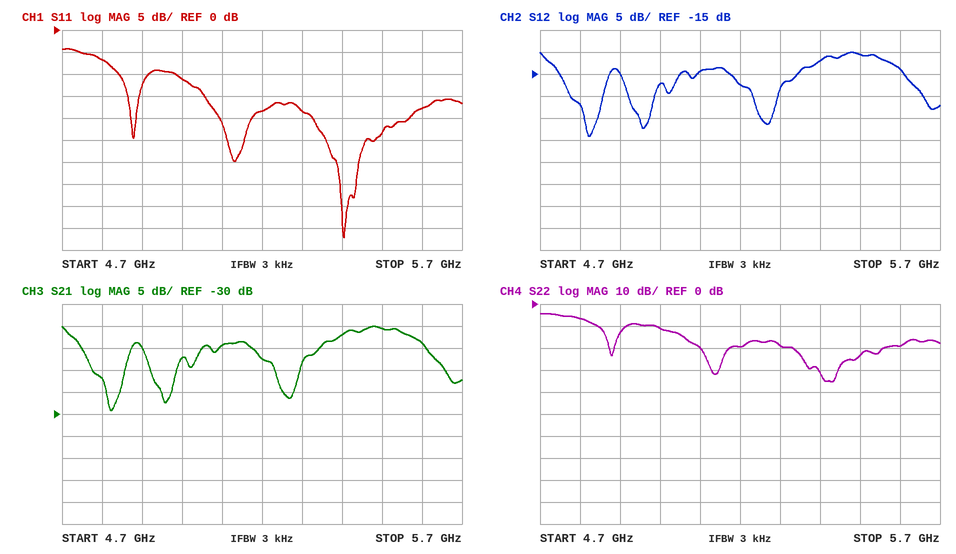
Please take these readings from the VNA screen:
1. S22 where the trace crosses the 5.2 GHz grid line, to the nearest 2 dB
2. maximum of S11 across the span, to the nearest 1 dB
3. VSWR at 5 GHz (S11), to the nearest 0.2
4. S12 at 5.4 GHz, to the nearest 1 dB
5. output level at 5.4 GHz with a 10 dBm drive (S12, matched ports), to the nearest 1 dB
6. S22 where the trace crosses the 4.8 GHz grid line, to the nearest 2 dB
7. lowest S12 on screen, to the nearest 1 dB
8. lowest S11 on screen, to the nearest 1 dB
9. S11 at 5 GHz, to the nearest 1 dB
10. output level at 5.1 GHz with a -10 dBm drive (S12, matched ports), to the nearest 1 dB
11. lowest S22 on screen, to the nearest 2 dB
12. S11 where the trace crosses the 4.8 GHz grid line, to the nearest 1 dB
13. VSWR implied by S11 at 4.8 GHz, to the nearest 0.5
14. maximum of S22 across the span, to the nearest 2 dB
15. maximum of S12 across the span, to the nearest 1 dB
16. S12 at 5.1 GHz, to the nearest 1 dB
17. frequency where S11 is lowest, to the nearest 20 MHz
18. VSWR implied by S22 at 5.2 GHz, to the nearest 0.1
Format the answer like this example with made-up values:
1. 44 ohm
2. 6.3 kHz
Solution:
1. -20 dB
2. -4 dB
3. 1.8
4. -12 dB
5. -2 dBm
6. -6 dB
7. -29 dB
8. -47 dB
9. -11 dB
10. -24 dBm
11. -36 dB
12. -7 dB
13. 2.5
14. -4 dB
15. -10 dB
16. -14 dB
17. 5.40 GHz
18. 1.2
